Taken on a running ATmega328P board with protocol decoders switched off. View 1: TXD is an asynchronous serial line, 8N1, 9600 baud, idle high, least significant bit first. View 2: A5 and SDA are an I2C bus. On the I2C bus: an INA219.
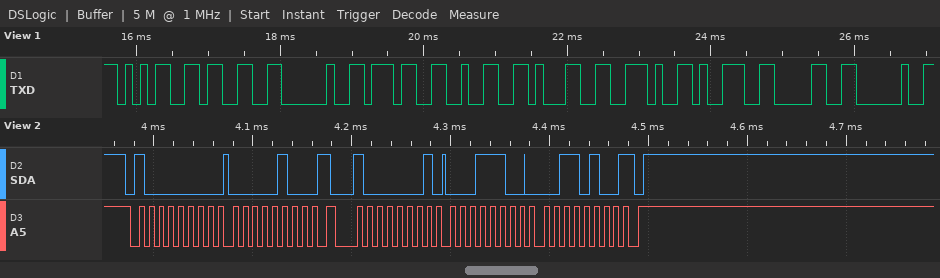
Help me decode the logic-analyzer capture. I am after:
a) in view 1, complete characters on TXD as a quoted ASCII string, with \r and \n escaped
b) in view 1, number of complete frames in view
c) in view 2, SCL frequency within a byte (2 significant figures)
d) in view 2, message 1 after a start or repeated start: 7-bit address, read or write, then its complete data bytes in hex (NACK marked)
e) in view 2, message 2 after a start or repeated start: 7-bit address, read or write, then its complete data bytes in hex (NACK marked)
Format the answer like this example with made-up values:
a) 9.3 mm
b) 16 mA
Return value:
a) "53 721.90 "
b) 10
c) 100 kHz
d) 0x40 write: 04
e) 0x40 read: 1C 34 NACK
